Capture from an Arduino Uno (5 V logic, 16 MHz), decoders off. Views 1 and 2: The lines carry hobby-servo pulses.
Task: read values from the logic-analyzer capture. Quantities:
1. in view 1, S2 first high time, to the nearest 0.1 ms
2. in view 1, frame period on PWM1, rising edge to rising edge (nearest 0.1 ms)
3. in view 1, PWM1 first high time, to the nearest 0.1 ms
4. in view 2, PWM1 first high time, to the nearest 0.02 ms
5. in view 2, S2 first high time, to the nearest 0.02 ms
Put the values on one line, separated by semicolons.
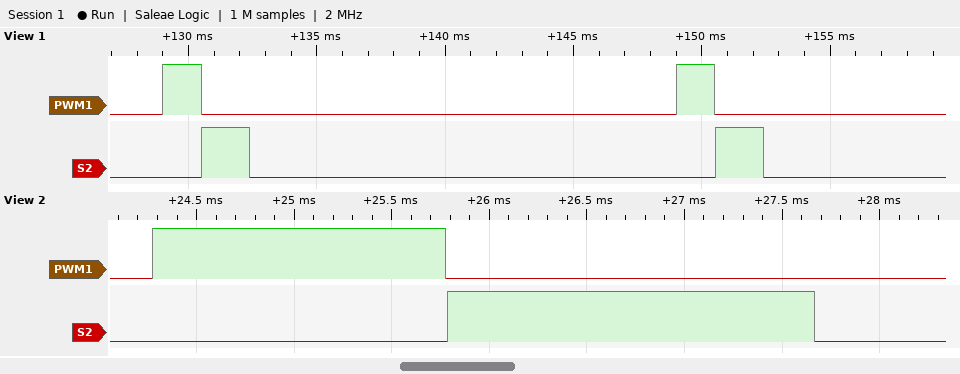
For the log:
1.9 ms; 20.0 ms; 1.5 ms; 1.50 ms; 1.88 ms
